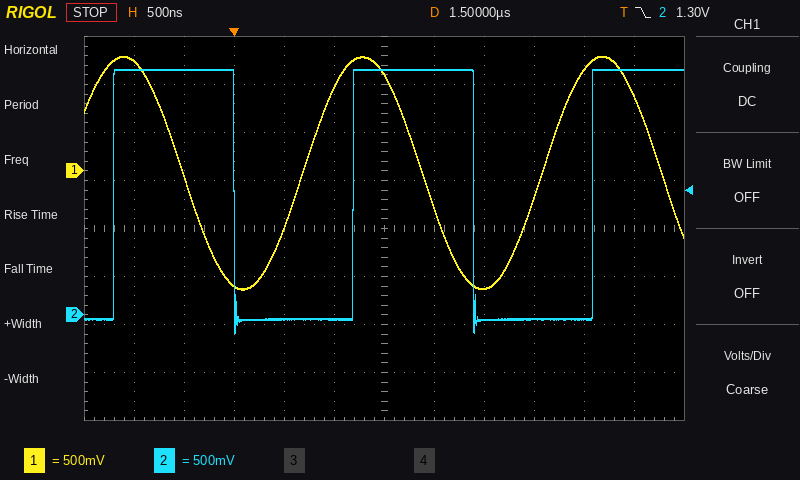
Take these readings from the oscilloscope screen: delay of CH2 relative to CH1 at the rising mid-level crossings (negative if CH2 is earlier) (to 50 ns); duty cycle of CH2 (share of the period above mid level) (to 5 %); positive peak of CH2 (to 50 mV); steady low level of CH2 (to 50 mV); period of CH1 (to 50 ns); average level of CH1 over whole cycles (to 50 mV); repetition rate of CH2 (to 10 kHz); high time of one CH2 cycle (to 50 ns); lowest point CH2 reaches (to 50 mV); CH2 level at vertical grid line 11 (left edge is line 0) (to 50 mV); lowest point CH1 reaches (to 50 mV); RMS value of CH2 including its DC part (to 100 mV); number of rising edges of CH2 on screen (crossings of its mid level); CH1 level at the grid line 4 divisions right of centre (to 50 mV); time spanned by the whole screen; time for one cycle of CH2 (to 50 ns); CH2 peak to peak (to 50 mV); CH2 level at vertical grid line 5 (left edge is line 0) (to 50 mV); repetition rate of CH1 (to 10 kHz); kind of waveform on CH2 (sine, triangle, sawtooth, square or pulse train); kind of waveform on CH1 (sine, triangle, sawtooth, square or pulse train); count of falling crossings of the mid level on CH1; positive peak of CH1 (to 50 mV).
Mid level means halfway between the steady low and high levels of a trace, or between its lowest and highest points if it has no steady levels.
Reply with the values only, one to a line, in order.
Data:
+500 ns
50 %
2.55 V
-50 mV
2.40 µs
0 mV
420 kHz
1.20 µs
-200 mV
2.55 V
-1.25 V
1.8 V
3
1.05 V
6 µs
2.40 µs
2.75 V
-50 mV
420 kHz
square
sine
3
1.20 V
